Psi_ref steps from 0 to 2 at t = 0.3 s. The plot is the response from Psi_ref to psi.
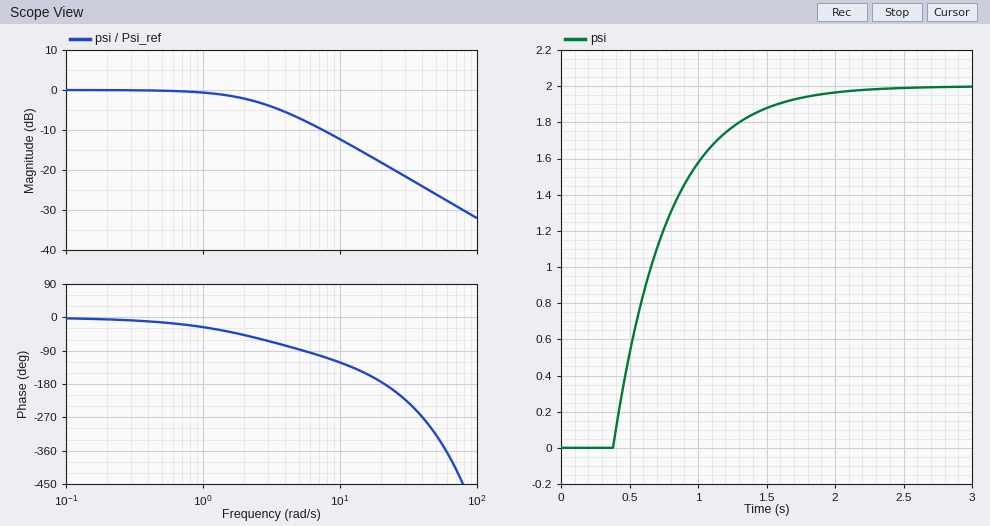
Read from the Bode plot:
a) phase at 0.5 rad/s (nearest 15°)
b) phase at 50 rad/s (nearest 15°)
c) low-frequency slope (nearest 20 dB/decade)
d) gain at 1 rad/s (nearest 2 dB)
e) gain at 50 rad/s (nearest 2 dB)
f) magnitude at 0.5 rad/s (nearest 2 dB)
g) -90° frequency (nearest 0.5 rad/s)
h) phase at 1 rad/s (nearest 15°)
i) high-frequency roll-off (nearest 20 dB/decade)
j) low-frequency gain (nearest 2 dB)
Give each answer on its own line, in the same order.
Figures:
-15°
-315°
0 dB/decade
0 dB
-26 dB
0 dB
5.5 rad/s
-30°
-20 dB/decade
0 dB
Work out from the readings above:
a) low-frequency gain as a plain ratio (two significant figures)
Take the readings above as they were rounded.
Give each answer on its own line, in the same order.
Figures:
1.0
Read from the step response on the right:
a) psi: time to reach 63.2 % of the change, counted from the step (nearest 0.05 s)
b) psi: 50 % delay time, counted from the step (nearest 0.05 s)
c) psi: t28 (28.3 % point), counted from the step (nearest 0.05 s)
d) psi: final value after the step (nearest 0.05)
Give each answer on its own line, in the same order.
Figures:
0.50 s
0.35 s
0.20 s
2.00
